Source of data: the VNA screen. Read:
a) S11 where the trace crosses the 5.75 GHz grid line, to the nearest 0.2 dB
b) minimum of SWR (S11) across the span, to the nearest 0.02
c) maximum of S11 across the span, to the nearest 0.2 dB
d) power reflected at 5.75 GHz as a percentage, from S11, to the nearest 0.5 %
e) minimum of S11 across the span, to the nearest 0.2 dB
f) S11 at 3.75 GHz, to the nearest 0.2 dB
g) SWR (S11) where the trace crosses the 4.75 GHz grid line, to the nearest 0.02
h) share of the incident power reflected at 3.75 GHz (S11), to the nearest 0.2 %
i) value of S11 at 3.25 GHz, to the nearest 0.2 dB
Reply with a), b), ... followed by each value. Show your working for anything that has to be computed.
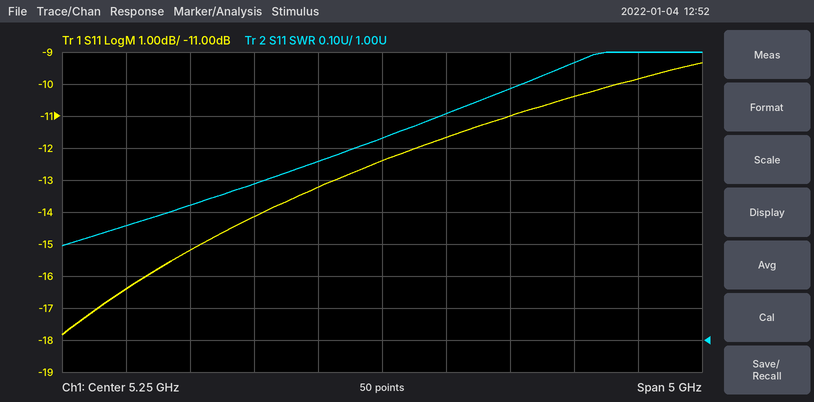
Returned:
a) -11.6 dB
b) 1.30
c) -9.4 dB
d) 10^(-11.6/10) ≈ 6.92 %, so 7.0 % to the nearest 0.5 %
e) -17.8 dB
f) -15.2 dB
g) 1.56
h) 10^(-15.2/10) ≈ 3.0 %
i) -16.4 dB
